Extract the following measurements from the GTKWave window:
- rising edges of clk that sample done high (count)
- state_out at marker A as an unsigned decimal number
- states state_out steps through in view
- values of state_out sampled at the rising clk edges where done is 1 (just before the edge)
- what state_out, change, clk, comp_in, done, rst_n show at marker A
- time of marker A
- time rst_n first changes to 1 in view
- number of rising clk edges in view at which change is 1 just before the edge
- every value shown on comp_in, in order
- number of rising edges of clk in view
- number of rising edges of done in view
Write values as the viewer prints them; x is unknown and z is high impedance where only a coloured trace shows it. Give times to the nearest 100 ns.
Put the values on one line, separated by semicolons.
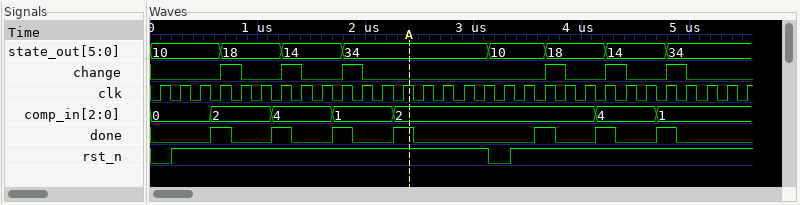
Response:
7; 52; 10, 18, 14, 34, 10, 18, 14, 34; 10, 18, 14, 34, 10, 18, 14; state_out=34, change=0, clk=1, comp_in=2, done=1, rst_n=1; 2400 ns; 200 ns; 6; 0, 2, 4, 1, 2, 4, 1; 30; 7
